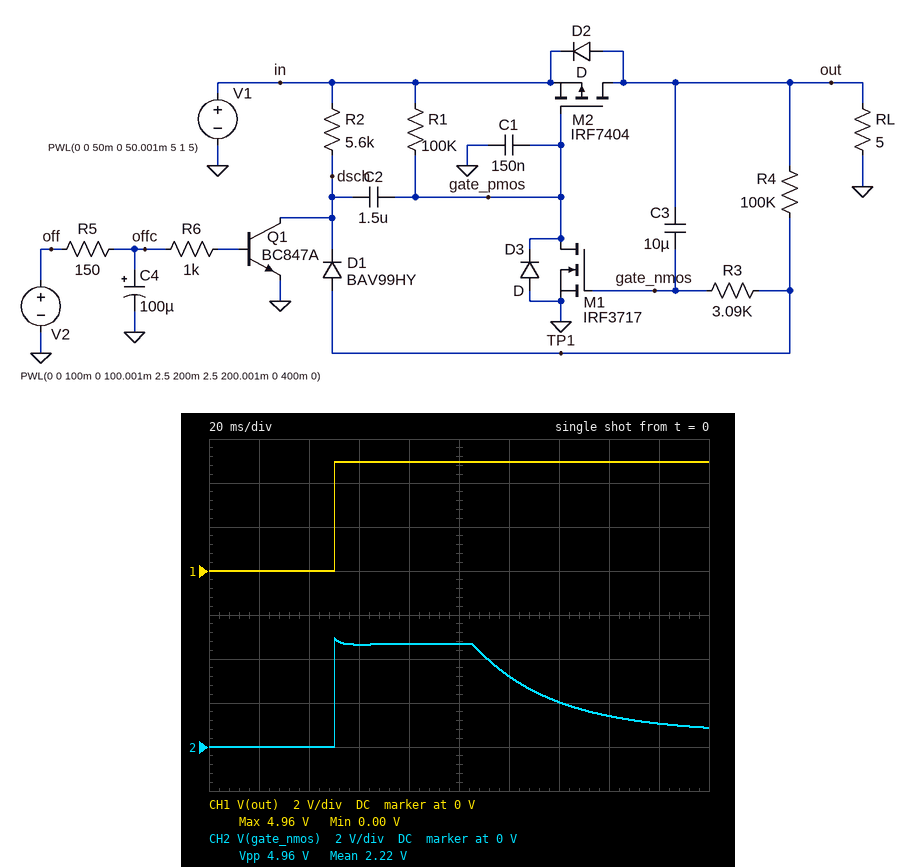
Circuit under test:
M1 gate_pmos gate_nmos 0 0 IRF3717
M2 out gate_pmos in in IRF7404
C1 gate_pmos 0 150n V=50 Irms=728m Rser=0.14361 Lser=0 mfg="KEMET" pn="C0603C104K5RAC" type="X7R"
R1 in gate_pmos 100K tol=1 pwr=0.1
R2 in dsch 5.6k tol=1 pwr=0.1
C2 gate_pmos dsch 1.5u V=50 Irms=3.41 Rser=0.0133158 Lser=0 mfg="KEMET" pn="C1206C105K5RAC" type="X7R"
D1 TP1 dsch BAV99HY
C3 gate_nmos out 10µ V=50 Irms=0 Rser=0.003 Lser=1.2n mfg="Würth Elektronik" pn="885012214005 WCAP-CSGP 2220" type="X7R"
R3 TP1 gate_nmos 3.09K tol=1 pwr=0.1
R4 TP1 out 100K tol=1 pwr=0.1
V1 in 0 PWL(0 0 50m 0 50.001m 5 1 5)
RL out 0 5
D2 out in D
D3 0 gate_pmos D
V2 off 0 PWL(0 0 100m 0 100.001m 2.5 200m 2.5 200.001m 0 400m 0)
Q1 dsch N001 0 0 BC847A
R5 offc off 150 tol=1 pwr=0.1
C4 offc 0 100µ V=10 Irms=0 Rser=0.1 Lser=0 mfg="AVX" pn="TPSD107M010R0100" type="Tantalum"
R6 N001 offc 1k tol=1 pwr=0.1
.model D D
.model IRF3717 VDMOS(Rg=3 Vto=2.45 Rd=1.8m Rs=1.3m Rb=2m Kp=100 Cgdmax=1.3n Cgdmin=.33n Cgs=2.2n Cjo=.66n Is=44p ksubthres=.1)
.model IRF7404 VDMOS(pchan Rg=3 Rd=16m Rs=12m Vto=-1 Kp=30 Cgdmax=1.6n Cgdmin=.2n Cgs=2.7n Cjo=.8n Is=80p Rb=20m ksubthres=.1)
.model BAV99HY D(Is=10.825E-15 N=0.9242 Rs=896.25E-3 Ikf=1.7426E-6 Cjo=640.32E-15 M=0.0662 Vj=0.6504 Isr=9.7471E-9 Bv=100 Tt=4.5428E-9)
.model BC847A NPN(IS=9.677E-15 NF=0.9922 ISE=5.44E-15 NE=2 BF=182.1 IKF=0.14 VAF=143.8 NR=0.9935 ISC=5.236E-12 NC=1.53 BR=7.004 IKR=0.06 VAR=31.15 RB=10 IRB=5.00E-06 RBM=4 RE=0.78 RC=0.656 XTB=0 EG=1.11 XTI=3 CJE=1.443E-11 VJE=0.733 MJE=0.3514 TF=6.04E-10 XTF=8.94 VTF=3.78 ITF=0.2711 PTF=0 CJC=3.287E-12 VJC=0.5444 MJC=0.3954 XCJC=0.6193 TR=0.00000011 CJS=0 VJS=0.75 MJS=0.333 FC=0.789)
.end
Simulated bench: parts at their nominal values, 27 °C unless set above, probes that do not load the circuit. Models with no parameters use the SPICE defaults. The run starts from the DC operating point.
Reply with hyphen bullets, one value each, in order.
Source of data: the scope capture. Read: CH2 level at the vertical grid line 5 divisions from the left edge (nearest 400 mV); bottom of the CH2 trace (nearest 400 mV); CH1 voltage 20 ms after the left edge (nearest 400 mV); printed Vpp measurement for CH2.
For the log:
- 4.8 V
- 0 V
- 0 V
- 4.96 V
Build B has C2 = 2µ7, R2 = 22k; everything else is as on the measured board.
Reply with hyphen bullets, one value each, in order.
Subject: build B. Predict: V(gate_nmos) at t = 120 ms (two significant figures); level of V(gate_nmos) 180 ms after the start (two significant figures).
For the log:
- 3.0 V
- 1.0 V
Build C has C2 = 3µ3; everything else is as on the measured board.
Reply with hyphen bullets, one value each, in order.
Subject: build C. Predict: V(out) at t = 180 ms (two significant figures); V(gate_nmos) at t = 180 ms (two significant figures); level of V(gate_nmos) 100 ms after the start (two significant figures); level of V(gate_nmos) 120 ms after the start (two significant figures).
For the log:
- 5.0 V
- 1.0 V
- 4.4 V
- 3.1 V
